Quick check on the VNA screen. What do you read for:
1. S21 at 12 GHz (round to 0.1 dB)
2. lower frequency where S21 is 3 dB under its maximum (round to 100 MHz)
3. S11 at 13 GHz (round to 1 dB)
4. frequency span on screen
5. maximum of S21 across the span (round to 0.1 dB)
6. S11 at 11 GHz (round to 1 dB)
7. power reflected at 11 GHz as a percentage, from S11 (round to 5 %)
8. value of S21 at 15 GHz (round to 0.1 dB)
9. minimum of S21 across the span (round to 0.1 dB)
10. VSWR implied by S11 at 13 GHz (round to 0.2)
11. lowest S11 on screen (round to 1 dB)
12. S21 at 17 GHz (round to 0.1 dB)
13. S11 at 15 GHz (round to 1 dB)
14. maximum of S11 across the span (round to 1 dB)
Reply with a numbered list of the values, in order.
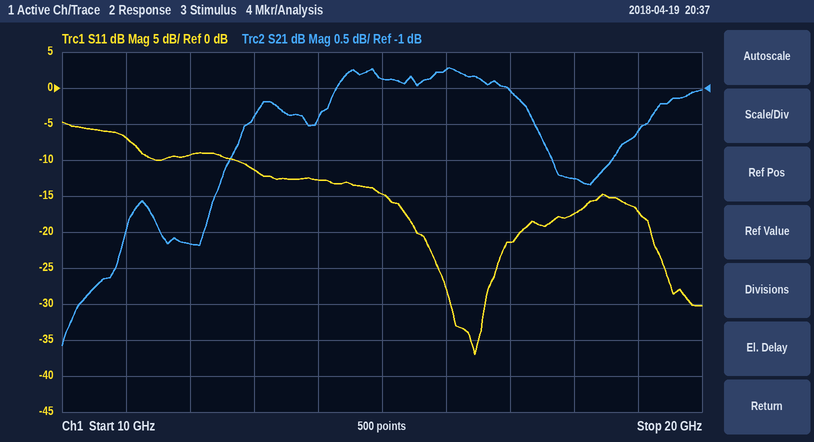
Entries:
1. -3.2 dB
2. 10.6 GHz
3. -11 dB
4. 10 GHz
5. -0.7 dB
6. -7 dB
7. 20 %
8. -0.9 dB
9. -4.6 dB
10. 1.8
11. -37 dB
12. -1.0 dB
13. -15 dB
14. -5 dB
